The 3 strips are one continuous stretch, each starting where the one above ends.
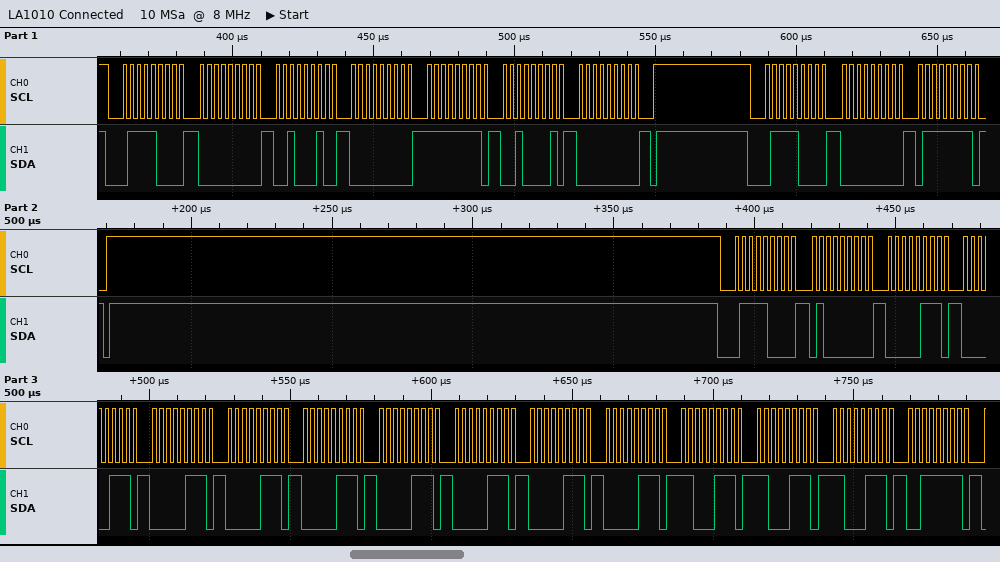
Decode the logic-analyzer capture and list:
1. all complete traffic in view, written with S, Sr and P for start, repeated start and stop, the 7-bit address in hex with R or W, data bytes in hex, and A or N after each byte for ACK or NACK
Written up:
S 3CW A 00 A 22 A 00 A FF A 21 A 00 A P S 3CW A 00 A 7F A P S 3CW A 40 A 07 A 07 A 07 A 07 A 07 A 07 A 07 A 07 A 07 A C7 A C7 A C7 A 3F A
